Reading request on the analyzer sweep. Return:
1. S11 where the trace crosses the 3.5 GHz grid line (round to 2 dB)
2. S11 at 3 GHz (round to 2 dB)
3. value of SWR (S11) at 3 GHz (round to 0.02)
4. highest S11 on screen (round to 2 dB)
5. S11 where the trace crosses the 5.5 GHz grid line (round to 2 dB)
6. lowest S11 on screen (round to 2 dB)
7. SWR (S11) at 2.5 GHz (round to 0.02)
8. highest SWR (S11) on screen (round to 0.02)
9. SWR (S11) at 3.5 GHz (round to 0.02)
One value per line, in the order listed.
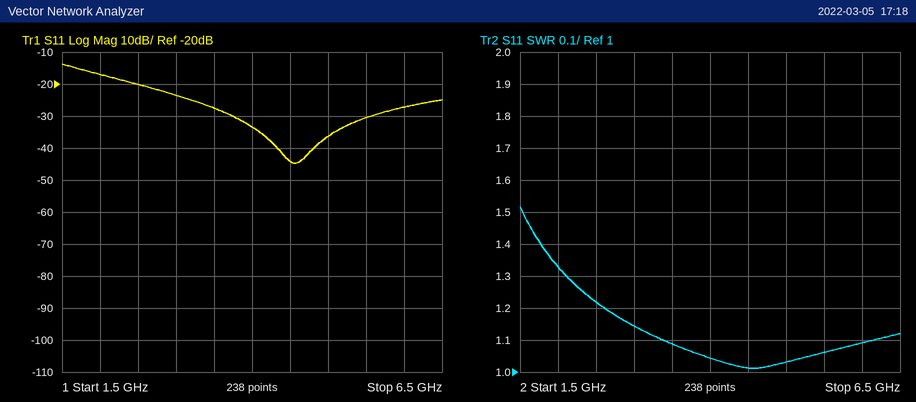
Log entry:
-28 dB
-24 dB
1.14
-14 dB
-30 dB
-44 dB
1.22
1.52
1.08
